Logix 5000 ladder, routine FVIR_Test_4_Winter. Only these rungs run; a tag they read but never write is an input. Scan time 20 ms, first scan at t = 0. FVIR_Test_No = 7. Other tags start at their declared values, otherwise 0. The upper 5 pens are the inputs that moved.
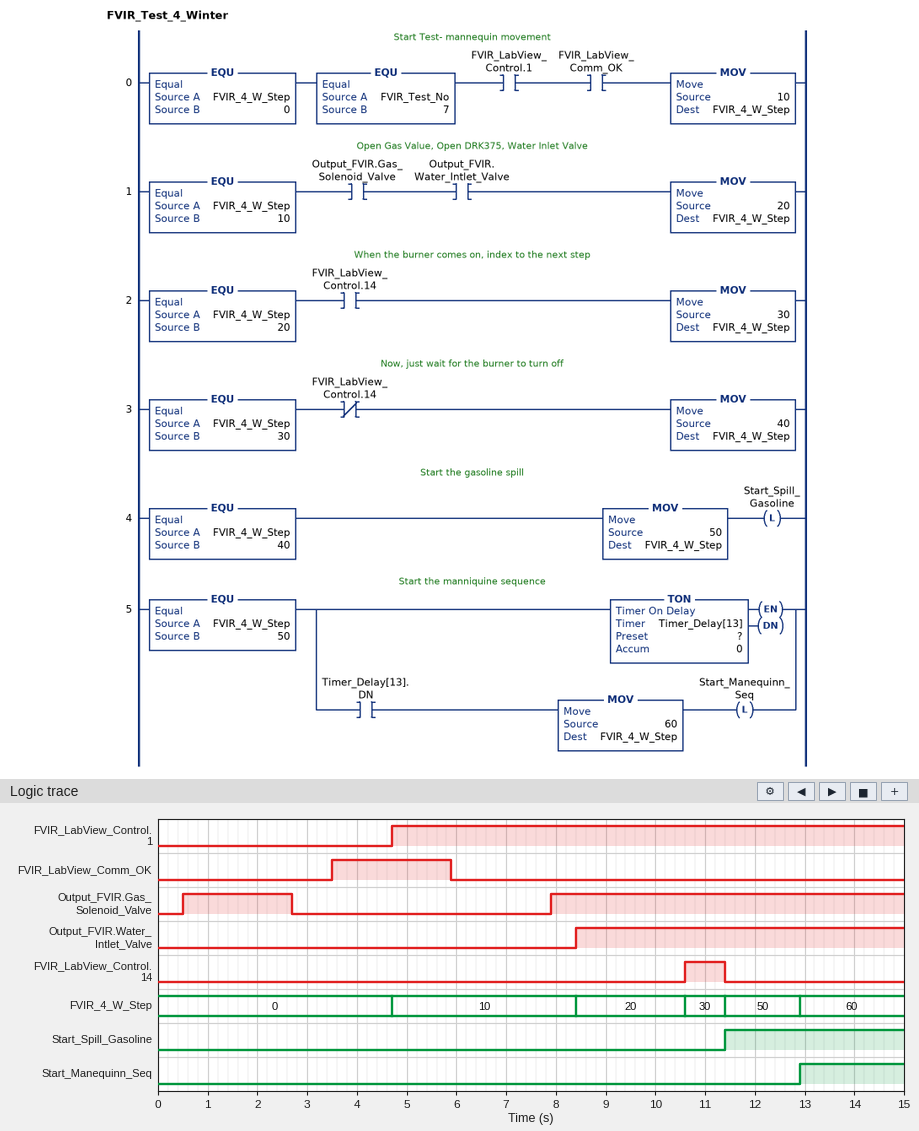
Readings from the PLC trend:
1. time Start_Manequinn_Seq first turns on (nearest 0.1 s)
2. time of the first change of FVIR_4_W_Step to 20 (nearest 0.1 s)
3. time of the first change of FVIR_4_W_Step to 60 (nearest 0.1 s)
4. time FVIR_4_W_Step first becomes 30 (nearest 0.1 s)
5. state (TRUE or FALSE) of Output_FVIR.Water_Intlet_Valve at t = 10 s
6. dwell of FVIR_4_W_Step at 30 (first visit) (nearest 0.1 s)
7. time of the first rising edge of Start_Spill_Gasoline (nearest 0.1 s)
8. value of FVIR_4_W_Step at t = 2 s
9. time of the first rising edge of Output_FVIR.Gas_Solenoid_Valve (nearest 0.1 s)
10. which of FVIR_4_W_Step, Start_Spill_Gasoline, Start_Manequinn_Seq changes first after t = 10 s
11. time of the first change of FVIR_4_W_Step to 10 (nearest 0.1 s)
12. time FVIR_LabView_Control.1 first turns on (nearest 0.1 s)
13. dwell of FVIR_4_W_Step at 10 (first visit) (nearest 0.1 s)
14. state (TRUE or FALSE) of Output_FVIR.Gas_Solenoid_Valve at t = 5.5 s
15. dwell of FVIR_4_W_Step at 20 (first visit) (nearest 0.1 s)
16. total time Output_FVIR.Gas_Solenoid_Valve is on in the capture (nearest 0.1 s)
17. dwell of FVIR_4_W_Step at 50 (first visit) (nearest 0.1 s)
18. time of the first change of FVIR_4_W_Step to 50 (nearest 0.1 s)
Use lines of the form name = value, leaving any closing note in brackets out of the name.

time Start_Manequinn_Seq first turns on = 12.9 s
time of the first change of FVIR_4_W_Step to 20 = 8.4 s
time of the first change of FVIR_4_W_Step to 60 = 12.9 s
time FVIR_4_W_Step first becomes 30 = 10.6 s
state (TRUE or FALSE) of Output_FVIR.Water_Intlet_Valve at t = 10 s = TRUE
dwell of FVIR_4_W_Step at 30 (first visit) = 0.8 s
time of the first rising edge of Start_Spill_Gasoline = 11.4 s
value of FVIR_4_W_Step at t = 2 s = 0
time of the first rising edge of Output_FVIR.Gas_Solenoid_Valve = 0.5 s
which of FVIR_4_W_Step, Start_Spill_Gasoline, Start_Manequinn_Seq changes first after t = 10 s = FVIR_4_W_Step
time of the first change of FVIR_4_W_Step to 10 = 4.7 s
time FVIR_LabView_Control.1 first turns on = 4.7 s
dwell of FVIR_4_W_Step at 10 (first visit) = 3.7 s
state (TRUE or FALSE) of Output_FVIR.Gas_Solenoid_Valve at t = 5.5 s = FALSE
dwell of FVIR_4_W_Step at 20 (first visit) = 2.2 s
total time Output_FVIR.Gas_Solenoid_Valve is on in the capture = 9.3 s
dwell of FVIR_4_W_Step at 50 (first visit) = 1.5 s
time of the first change of FVIR_4_W_Step to 50 = 11.4 s
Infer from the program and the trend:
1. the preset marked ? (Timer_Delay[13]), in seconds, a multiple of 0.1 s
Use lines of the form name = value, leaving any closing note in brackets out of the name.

the preset marked ? (Timer_Delay[13]), in seconds, a multiple of 0.1 s = 1.5 s
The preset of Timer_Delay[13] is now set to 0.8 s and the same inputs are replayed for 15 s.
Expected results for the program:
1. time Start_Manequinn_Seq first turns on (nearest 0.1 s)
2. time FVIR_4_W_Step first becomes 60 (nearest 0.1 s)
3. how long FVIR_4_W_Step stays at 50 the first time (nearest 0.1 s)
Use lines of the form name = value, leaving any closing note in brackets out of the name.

time Start_Manequinn_Seq first turns on = 12.2 s
time FVIR_4_W_Step first becomes 60 = 12.2 s
how long FVIR_4_W_Step stays at 50 the first time = 0.8 s
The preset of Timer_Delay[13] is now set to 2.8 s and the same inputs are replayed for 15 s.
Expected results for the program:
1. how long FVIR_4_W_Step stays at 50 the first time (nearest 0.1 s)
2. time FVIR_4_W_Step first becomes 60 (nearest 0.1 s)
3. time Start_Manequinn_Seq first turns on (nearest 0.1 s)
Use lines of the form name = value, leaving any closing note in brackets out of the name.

how long FVIR_4_W_Step stays at 50 the first time = 2.8 s
time FVIR_4_W_Step first becomes 60 = 14.2 s
time Start_Manequinn_Seq first turns on = 14.2 s
